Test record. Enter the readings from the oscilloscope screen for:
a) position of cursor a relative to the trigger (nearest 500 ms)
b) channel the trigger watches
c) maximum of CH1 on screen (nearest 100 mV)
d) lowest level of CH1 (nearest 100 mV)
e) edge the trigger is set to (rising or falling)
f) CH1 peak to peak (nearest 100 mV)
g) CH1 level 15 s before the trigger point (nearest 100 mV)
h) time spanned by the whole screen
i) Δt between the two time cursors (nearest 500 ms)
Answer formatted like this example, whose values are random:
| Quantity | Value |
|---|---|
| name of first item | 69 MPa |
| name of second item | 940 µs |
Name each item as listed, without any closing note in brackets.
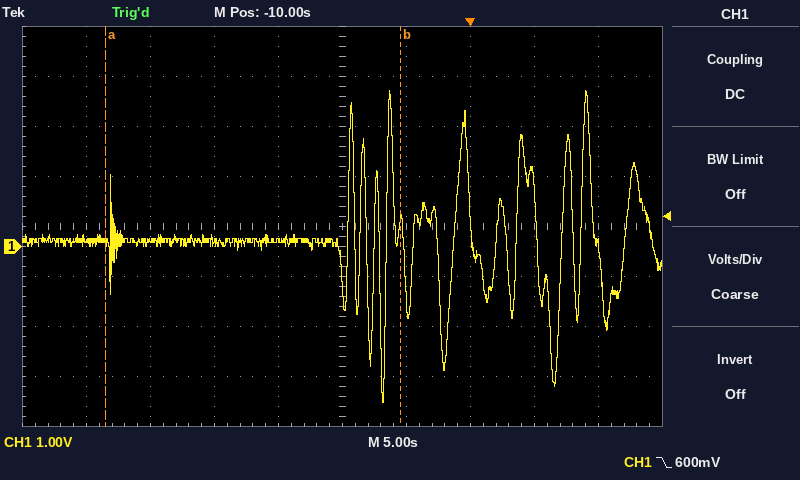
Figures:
| Quantity | Value |
|---|---|
| position of cursor a relative to the trigger | -28.5 s |
| channel the trigger watches | CH1 |
| maximum of CH1 on screen | 3.1 V |
| lowest level of CH1 | -3.1 V |
| edge the trigger is set to | falling |
| CH1 peak to peak | 6.2 V |
| CH1 level 15 s before the trigger point | 100 mV |
| time spanned by the whole screen | 50 s |
| Δt between the two time cursors | 23.0 s |
